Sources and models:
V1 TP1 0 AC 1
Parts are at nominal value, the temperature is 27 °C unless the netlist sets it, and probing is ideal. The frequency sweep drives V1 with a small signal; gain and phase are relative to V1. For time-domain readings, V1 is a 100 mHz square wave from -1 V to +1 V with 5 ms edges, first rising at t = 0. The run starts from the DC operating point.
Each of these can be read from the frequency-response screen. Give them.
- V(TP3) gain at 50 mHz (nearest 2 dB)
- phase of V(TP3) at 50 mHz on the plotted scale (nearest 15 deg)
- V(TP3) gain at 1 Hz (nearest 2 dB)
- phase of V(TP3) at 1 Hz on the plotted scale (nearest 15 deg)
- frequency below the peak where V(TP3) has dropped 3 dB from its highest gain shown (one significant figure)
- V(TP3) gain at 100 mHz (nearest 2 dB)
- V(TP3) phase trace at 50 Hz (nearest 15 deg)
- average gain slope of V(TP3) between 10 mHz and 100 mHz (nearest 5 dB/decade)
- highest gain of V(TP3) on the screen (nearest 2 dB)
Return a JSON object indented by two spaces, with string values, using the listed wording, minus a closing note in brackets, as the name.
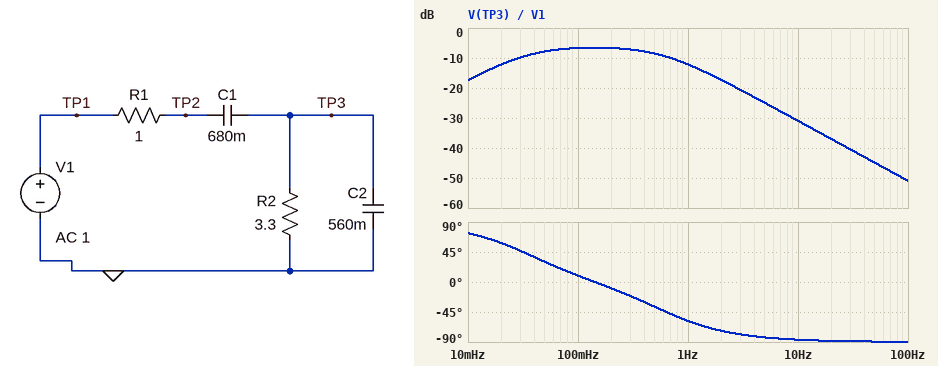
{
  "V(TP3) gain at 50 mHz": "-8 dB",
  "phase of V(TP3) at 50 mHz on the plotted scale": "30 deg",
  "V(TP3) gain at 1 Hz": "-12 dB",
  "phase of V(TP3) at 1 Hz on the plotted scale": "-60 deg",
  "frequency below the peak where V(TP3) has dropped 3 dB from its highest gain shown": "30 mHz",
  "V(TP3) gain at 100 mHz": "-6 dB",
  "V(TP3) phase trace at 50 Hz": "-90 deg",
  "average gain slope of V(TP3) between 10 mHz and 100 mHz": "10 dB/decade",
  "highest gain of V(TP3) on the screen": "-6 dB"
}
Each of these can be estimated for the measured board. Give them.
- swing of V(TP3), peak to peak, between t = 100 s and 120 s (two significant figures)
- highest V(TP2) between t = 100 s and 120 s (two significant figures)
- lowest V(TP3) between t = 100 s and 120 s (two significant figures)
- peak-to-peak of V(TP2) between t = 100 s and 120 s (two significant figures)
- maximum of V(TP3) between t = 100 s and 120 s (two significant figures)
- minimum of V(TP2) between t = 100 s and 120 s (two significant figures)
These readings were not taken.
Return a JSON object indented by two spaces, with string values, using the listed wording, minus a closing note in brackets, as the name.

{
  "swing of V(TP3), peak to peak, between t = 100 s and 120 s": "1.2 V",
  "highest V(TP2) between t = 100 s and 120 s": "950 mV",
  "lowest V(TP3) between t = 100 s and 120 s": "-610 mV",
  "peak-to-peak of V(TP2) between t = 100 s and 120 s": "1.9 V",
  "maximum of V(TP3) between t = 100 s and 120 s": "610 mV",
  "minimum of V(TP2) between t = 100 s and 120 s": "-950 mV"
}
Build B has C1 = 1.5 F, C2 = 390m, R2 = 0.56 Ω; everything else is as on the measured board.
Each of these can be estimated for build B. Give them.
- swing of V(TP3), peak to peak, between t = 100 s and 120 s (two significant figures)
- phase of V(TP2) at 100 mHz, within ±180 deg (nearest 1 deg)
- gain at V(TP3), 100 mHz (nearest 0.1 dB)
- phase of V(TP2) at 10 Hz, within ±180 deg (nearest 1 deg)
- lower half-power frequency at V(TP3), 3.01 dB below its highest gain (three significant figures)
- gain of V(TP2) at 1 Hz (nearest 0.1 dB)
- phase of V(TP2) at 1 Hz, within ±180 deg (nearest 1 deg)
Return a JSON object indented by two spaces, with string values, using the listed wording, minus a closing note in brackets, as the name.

{
  "swing of V(TP3), peak to peak, between t = 100 s and 120 s": "1.0 V",
  "phase of V(TP2) at 100 mHz, within ±180 deg": "-28 deg",
  "gain at V(TP3), 100 mHz": "-10.8 dB",
  "phase of V(TP2) at 10 Hz, within ±180 deg": "-84 deg",
  "lower half-power frequency at V(TP3), 3.01 dB below its highest gain": "59.4 mHz",
  "gain of V(TP2) at 1 Hz": "-9.5 dB",
  "phase of V(TP2) at 1 Hz, within ±180 deg": "-45 deg"
}
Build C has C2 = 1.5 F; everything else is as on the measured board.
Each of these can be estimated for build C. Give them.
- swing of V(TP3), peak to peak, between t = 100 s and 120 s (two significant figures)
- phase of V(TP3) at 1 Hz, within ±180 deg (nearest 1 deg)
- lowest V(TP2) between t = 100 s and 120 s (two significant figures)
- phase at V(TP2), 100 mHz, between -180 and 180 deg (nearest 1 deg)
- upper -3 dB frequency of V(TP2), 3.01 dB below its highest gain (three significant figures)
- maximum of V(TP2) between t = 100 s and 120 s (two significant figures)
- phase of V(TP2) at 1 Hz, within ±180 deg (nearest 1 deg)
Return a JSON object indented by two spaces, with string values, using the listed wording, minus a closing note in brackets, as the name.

{
  "swing of V(TP3), peak to peak, between t = 100 s and 120 s": "650 mV",
  "phase of V(TP3) at 1 Hz, within ±180 deg": "-69 deg",
  "lowest V(TP2) between t = 100 s and 120 s": "-980 mV",
  "phase at V(TP2), 100 mHz, between -180 and 180 deg": "-16 deg",
  "upper -3 dB frequency of V(TP2), 3.01 dB below its highest gain": "329 mHz",
  "maximum of V(TP2) between t = 100 s and 120 s": "980 mV",
  "phase of V(TP2) at 1 Hz, within ±180 deg": "-71 deg"
}
